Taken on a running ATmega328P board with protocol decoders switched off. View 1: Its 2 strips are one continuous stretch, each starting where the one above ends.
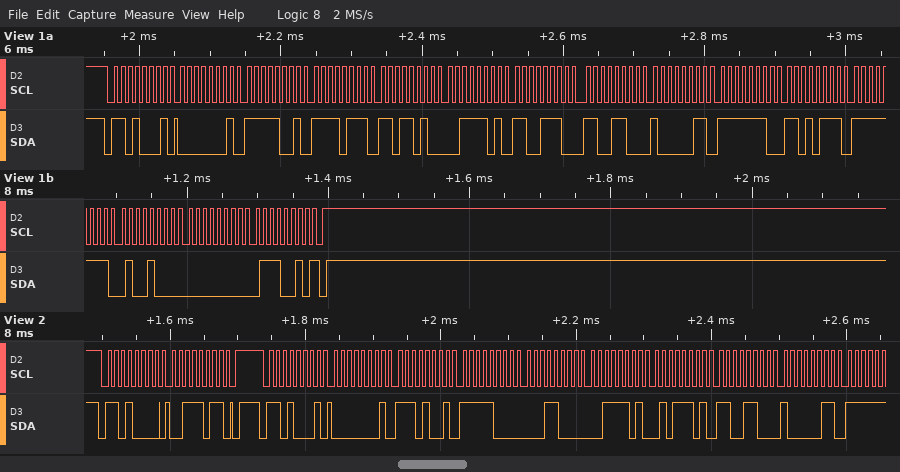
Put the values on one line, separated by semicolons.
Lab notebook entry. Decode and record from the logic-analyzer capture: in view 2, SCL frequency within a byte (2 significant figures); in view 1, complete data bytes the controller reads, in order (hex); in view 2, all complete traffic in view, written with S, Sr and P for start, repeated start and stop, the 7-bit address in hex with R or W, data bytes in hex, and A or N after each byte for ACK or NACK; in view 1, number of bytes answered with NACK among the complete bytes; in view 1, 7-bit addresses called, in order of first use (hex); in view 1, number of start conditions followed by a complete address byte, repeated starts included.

100 kHz; 01 F9 F7 DA 3D CE CC 83 FE D7 FF 48 00 72; S 68W A 3B A P S 68R A 01 A E9 A F8 A 18 A 3D A 5D A CC A 83 A; 1; 0x68; 1
